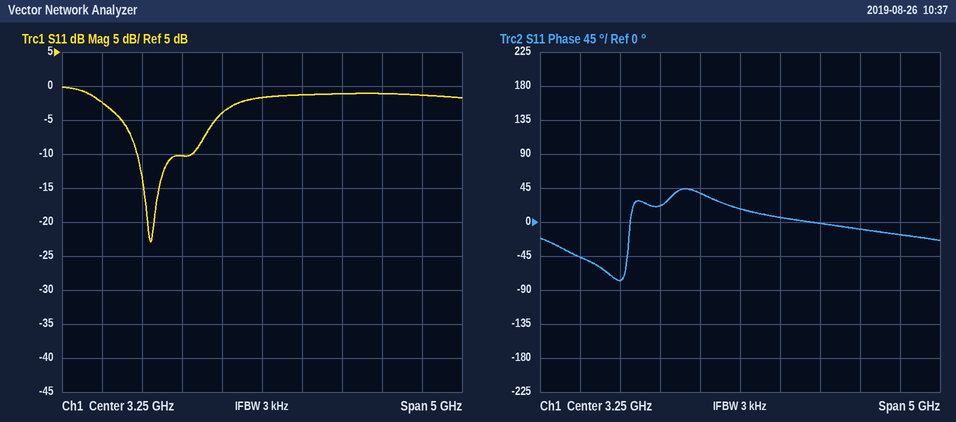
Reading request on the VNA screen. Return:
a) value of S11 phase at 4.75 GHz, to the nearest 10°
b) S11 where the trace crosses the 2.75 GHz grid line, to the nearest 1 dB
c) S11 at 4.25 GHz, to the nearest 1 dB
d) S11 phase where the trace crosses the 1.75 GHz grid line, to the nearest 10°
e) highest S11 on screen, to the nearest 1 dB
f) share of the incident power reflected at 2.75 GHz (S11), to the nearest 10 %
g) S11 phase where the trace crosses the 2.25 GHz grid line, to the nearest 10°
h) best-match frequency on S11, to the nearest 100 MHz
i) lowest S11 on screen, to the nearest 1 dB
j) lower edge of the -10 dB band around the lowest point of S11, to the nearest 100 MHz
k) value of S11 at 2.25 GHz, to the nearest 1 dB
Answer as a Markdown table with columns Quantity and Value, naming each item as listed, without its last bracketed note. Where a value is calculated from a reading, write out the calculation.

| Quantity | Value |
|---|---|
| value of S11 phase at 4.75 GHz, to the nearest 10° | -10° |
| S11 where the trace crosses the 2.75 GHz grid line, to the nearest 1 dB | -4 dB |
| S11 at 4.25 GHz, to the nearest 1 dB | -1 dB |
| S11 phase where the trace crosses the 1.75 GHz grid line, to the nearest 10° | -80° |
| highest S11 on screen, to the nearest 1 dB | 0 dB |
| share of the incident power reflected at 2.75 GHz (S11), to the nearest 10 % | 10^(-4/10) ≈ 40 % |
| S11 phase where the trace crosses the 2.25 GHz grid line, to the nearest 10° | 20° |
| best-match frequency on S11, to the nearest 100 MHz | 1.9 GHz |
| lowest S11 on screen, to the nearest 1 dB | -23 dB |
| lower edge of the -10 dB band around the lowest point of S11, to the nearest 100 MHz | 1.7 GHz |
| value of S11 at 2.25 GHz, to the nearest 1 dB | -10 dB |
